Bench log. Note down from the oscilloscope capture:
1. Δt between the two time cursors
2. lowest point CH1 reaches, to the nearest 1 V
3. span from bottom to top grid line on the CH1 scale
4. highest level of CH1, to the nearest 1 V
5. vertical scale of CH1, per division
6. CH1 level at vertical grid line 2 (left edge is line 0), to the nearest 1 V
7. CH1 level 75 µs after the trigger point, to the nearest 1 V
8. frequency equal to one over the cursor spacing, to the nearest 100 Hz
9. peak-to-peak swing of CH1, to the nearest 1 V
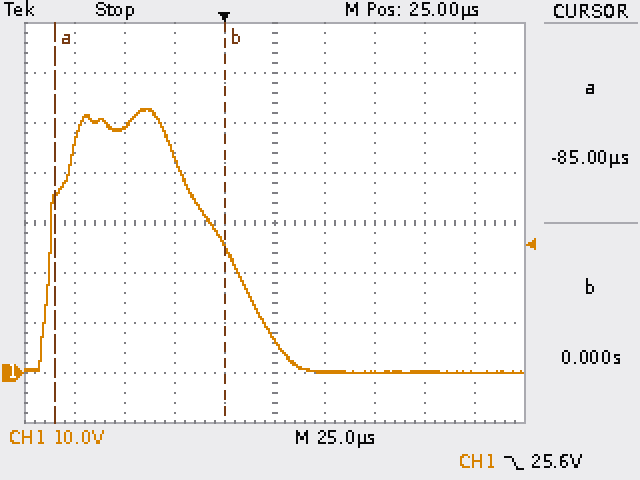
85.0 µs
0 V
80 V
53 V
10 V
49 V
0 V
11.8 kHz
53 V
